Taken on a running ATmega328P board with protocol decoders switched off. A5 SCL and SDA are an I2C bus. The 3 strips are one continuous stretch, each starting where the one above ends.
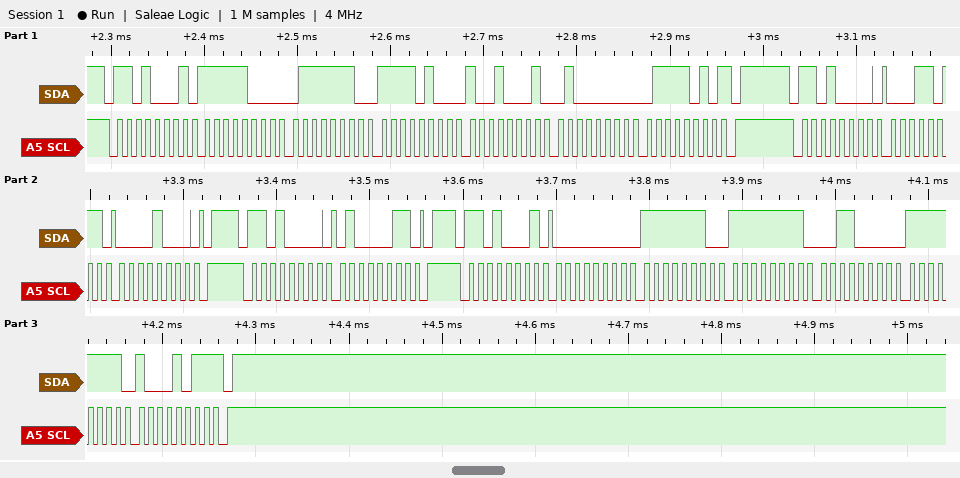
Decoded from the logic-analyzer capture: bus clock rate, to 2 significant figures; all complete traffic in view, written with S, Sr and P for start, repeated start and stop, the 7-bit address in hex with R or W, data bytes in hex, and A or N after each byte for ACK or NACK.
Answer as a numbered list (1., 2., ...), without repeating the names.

1. 100 kHz
2. S 68R A F8 A 7E A F4 A 91 A 40 A 7A N P S 68W A 1B A 08 A P S 68W A 43 A P S 68R A 00 A FE A FF A 30 A FF A 8B N P
